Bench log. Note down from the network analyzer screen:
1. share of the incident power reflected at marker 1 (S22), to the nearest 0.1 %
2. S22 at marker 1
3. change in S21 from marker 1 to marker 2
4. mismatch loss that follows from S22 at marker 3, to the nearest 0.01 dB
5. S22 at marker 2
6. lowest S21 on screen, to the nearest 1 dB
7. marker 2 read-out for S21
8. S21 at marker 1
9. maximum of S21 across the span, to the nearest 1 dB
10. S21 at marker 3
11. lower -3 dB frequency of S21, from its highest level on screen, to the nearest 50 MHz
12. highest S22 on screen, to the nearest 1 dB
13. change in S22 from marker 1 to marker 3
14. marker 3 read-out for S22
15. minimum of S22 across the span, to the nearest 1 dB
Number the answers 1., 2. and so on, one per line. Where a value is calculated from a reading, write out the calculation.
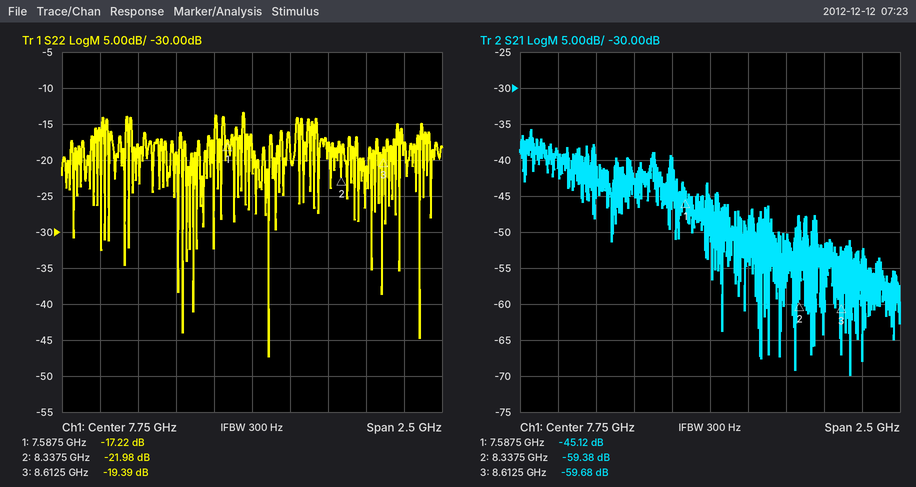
1. 10^(-17.22/10) ≈ 1.9 %
2. -17.22 dB
3. -59.38 − (-45.12) = -14.26 dB
4. −10 log10(1 − 10^(-19.39/10)) ≈ 0.05 dB
5. -21.98 dB
6. -70 dB
7. -59.38 dB
8. -45.12 dB
9. -36 dB
10. -59.68 dB
11. 6.55 GHz
12. -13 dB
13. -19.39 − (-17.22) = -2.17 dB
14. -19.39 dB
15. -47 dB
